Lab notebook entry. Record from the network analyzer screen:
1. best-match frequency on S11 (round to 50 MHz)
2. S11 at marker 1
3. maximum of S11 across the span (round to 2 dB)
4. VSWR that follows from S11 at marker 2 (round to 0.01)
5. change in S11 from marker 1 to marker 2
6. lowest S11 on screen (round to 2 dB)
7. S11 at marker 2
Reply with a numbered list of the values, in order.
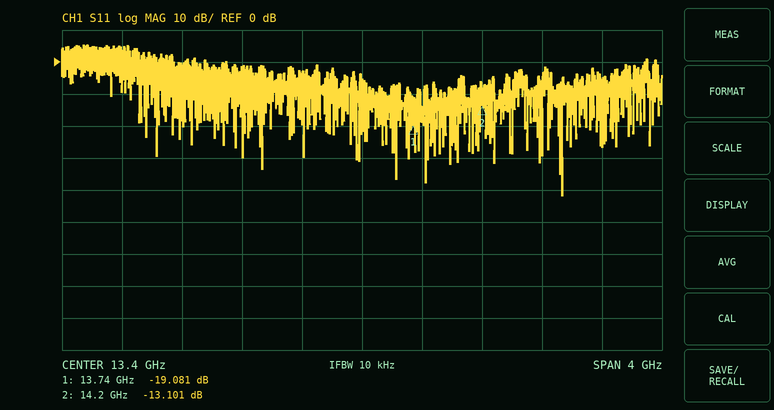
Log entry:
1. 14.75 GHz
2. -19.081 dB
3. 6 dB
4. 1.57
5. 5.980 dB
6. -42 dB
7. -13.101 dB
